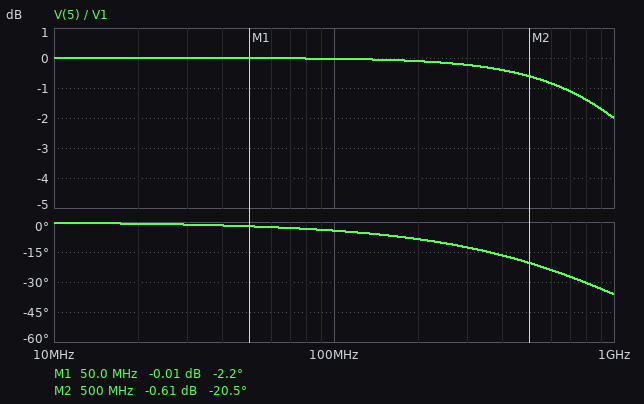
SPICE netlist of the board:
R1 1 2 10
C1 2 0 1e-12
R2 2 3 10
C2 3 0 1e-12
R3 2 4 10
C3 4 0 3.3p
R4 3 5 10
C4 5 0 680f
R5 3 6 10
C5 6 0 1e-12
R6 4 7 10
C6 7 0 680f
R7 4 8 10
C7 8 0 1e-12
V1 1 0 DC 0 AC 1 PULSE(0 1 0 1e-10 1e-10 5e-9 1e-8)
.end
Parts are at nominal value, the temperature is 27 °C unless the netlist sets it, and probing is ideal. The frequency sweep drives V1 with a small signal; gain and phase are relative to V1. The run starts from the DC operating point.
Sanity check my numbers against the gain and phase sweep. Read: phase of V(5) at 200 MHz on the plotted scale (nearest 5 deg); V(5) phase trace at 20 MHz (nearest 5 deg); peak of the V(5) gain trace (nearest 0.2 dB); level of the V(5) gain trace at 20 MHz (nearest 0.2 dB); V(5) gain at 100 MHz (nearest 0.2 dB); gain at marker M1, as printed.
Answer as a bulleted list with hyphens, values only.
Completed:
- -10 deg
- 0 deg
- 0 dB
- 0 dB
- 0 dB
- -0.01 dB
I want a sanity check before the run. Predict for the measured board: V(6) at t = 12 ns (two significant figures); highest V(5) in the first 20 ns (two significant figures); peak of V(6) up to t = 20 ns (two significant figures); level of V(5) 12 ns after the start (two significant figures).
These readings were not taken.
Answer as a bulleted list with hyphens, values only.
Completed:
- 1.0 V
- 1.0 V
- 1.0 V
- 1.0 V
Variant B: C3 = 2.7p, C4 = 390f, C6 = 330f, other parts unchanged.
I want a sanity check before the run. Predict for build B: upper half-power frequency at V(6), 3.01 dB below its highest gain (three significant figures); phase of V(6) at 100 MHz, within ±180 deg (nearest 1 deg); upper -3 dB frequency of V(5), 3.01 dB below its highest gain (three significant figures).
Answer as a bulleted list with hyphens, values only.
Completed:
- 1.54 GHz
- -4 deg
- 1.55 GHz
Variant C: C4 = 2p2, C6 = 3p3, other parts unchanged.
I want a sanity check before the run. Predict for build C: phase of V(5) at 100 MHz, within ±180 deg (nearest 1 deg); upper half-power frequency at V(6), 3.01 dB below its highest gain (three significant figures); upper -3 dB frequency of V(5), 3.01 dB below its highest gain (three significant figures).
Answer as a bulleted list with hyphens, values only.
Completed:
- -7 deg
- 856 MHz
- 846 MHz
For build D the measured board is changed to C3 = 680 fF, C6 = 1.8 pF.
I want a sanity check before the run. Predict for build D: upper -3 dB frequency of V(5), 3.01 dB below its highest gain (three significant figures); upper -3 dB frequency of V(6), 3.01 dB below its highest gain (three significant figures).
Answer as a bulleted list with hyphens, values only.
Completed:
- 1.55 GHz
- 1.54 GHz
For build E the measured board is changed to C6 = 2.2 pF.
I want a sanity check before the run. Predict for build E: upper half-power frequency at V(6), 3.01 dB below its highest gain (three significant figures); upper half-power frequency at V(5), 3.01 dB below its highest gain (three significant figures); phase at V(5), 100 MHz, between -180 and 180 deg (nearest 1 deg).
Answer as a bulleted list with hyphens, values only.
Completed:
- 1.13 GHz
- 1.14 GHz
- -5 deg
